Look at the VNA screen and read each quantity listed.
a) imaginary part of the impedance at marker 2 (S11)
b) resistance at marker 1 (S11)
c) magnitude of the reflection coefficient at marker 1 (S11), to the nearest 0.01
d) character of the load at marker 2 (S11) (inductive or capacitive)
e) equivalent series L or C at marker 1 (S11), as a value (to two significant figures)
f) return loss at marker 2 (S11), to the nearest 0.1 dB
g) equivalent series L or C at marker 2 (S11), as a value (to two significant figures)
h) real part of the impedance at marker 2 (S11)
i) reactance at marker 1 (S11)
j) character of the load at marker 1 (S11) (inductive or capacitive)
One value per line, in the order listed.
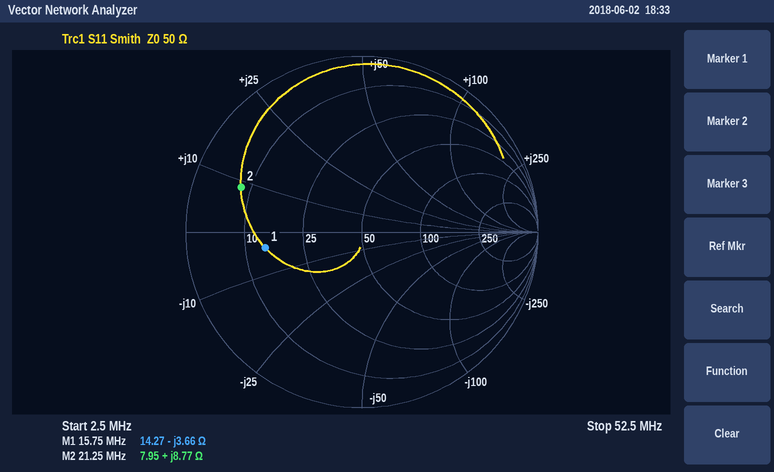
+8.77 Ω
14.27 Ω
0.56
inductive
2.8 nF
2.7 dB
66 nH
7.95 Ω
-3.66 Ω
capacitive
